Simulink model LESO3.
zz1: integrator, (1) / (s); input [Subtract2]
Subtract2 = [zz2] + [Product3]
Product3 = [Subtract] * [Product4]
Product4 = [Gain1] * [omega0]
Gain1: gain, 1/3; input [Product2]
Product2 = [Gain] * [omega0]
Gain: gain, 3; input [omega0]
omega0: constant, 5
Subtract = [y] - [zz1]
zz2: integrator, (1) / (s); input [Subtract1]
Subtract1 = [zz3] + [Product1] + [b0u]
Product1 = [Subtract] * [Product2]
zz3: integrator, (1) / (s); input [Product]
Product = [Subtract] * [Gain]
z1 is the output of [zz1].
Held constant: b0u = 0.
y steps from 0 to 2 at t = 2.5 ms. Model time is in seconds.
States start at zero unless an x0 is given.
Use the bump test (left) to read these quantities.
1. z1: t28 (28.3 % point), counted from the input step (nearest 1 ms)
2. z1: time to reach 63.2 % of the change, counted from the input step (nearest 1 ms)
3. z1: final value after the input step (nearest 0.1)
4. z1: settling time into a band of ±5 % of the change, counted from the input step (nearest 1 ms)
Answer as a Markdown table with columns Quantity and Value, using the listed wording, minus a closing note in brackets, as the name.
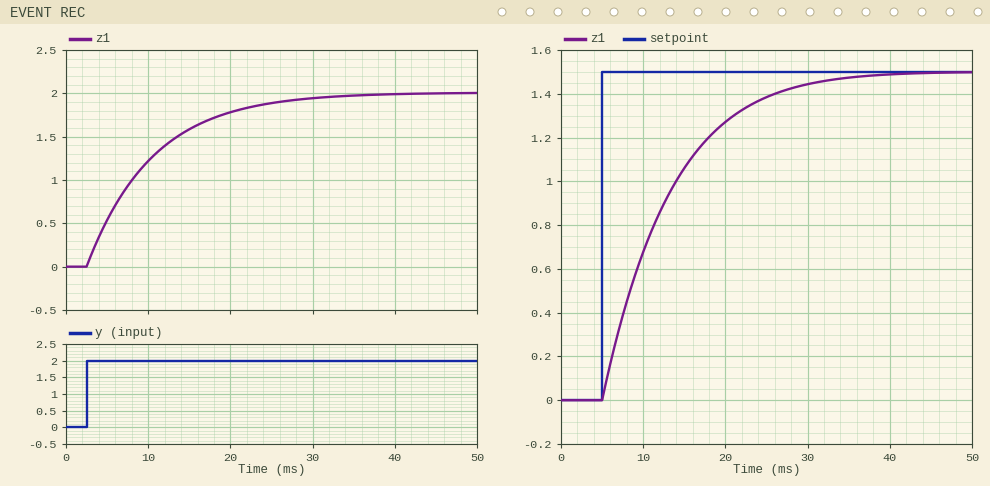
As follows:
| Quantity | Value |
|---|---|
| z1: t28 (28.3 % point), counted from the input step | 3 ms |
| z1: time to reach 63.2 % of the change, counted from the input step | 8 ms |
| z1: final value after the input step | 2.0 |
| z1: settling time into a band of ±5 % of the change, counted from the input step | 24 ms |
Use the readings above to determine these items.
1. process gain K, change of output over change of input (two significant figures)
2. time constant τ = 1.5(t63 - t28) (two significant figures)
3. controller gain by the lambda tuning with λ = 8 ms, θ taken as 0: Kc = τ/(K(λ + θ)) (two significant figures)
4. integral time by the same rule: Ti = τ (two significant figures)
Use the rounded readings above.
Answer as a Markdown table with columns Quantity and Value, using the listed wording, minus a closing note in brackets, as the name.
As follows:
| Quantity | Value |
|---|---|
| process gain K, change of output over change of input | 1.0 |
| time constant τ = 1.5(t63 - t28) | 7.5 ms |
| controller gain by the lambda tuning with λ = 8 ms, θ taken as 0: Kc = τ/(K(λ + θ)) | 0.94 |
| integral time by the same rule: Ti = τ | 7.5 ms |
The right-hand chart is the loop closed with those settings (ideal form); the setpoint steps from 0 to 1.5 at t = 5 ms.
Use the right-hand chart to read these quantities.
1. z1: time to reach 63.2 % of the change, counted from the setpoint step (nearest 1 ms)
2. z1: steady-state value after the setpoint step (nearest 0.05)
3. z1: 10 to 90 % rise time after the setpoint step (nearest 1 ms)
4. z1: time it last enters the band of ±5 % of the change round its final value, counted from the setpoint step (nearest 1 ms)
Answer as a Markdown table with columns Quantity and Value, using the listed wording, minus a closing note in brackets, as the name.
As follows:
| Quantity | Value |
|---|---|
| z1: time to reach 63.2 % of the change, counted from the setpoint step | 8 ms |
| z1: steady-state value after the setpoint step | 1.50 |
| z1: 10 to 90 % rise time after the setpoint step | 17 ms |
| z1: time it last enters the band of ±5 % of the change round its final value, counted from the setpoint step | 23 ms |
